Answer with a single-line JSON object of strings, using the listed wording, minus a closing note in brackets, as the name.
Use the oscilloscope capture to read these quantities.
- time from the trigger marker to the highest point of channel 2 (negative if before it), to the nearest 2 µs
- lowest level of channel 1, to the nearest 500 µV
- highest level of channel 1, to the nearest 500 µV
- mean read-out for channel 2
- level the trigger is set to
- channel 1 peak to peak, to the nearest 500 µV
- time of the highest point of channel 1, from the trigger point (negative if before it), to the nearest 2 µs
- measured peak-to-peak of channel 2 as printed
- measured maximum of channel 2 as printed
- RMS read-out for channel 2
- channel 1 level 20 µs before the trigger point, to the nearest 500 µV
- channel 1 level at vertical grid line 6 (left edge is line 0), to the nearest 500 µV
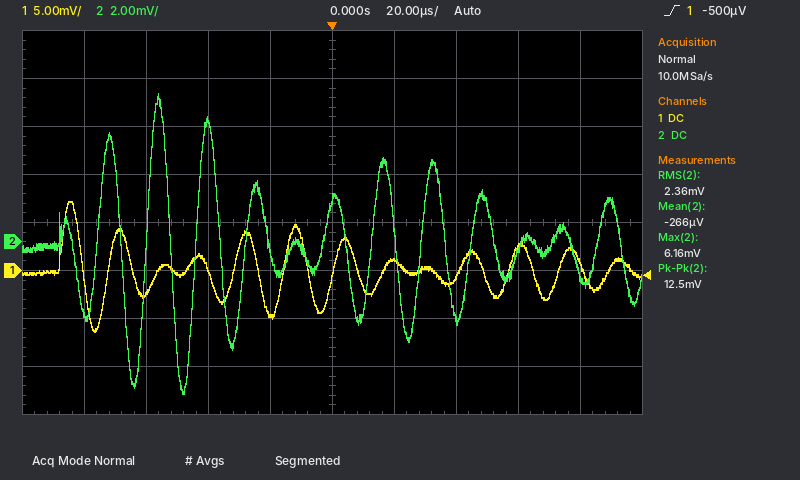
{"time from the trigger marker to the highest point of channel 2 (negative if before it), to the nearest 2 µs": "-56 µs", "lowest level of channel 1, to the nearest 500 µV": "-6.5 mV", "highest level of channel 1, to the nearest 500 µV": "7.0 mV", "mean read-out for channel 2": "-266 µV", "level the trigger is set to": "-500 µV", "channel 1 peak to peak, to the nearest 500 µV": "13.5 mV", "time of the highest point of channel 1, from the trigger point (negative if before it), to the nearest 2 µs": "-84 µs", "measured peak-to-peak of channel 2 as printed": "12.5 mV", "measured maximum of channel 2 as printed": "6.16 mV", "RMS read-out for channel 2": "2.36 mV", "channel 1 level 20 µs before the trigger point, to the nearest 500 µV": "-4.5 mV", "channel 1 level at vertical grid line 6 (left edge is line 0), to the nearest 500 µV": "1.0 mV"}
